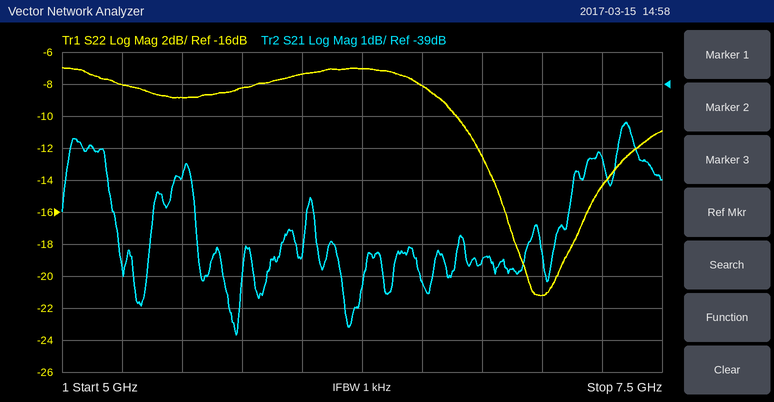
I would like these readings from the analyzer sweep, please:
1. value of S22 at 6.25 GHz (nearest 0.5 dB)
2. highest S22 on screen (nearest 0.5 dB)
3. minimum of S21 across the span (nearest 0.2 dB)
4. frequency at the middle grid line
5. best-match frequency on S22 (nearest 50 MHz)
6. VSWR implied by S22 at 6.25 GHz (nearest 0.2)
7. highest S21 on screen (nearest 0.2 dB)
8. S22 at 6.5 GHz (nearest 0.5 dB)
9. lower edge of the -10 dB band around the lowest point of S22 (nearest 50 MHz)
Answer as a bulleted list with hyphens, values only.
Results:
- -7.0 dB
- -7.0 dB
- -46.8 dB
- 6.25 GHz
- 7.00 GHz
- 2.6
- -40.2 dB
- -8.0 dB
- 6.65 GHz
